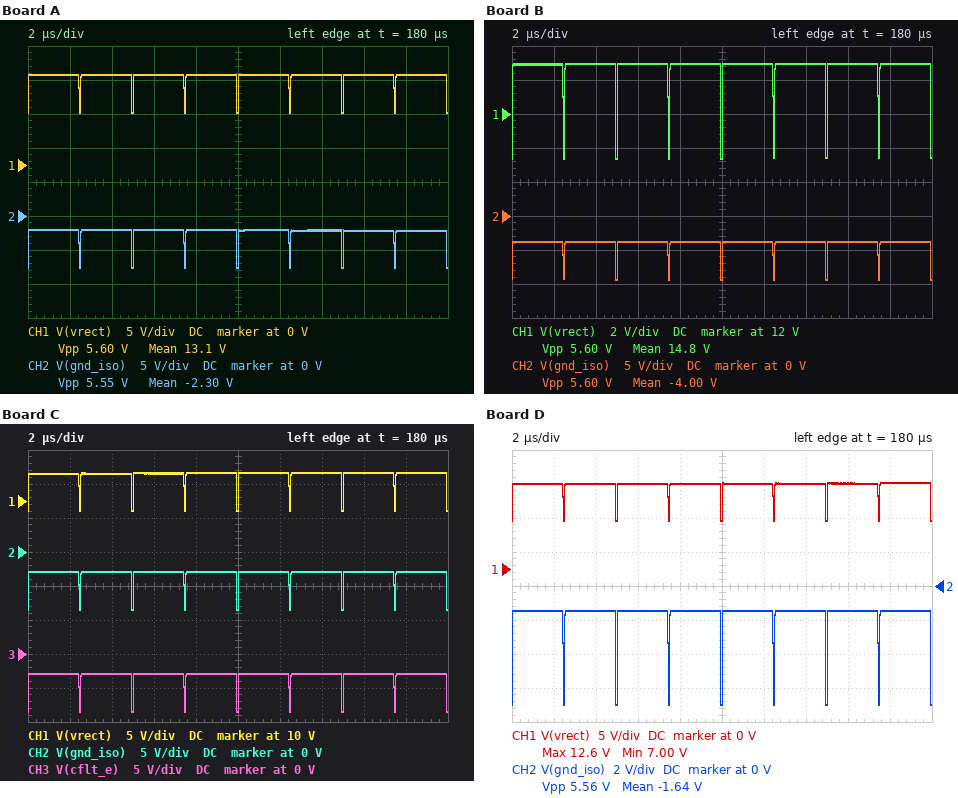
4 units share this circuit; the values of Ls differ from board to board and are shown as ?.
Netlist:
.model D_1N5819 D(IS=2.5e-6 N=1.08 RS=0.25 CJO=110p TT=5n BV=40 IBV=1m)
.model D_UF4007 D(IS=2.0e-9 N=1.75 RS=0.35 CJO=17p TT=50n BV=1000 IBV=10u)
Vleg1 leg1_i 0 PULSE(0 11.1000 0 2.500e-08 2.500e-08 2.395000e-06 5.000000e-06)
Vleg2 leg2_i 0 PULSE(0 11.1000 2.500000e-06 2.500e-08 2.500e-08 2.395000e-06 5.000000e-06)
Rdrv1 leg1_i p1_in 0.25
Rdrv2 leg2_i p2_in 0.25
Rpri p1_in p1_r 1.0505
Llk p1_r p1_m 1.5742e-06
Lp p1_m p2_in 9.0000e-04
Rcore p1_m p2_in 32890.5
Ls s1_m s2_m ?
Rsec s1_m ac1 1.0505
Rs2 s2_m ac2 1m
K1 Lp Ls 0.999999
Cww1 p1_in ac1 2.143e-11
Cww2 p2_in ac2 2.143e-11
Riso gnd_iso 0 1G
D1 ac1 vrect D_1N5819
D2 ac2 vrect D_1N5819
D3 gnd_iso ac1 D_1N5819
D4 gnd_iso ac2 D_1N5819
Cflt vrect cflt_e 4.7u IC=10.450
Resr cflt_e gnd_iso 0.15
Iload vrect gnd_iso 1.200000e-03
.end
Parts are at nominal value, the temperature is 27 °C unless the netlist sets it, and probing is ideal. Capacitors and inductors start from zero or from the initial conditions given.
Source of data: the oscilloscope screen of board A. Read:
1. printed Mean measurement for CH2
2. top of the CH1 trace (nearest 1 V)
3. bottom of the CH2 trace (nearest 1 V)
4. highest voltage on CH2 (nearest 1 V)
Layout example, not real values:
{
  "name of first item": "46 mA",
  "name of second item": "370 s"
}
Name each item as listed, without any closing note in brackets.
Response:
{
  "printed Mean measurement for CH2": "-2.30 V",
  "top of the CH1 trace": "13 V",
  "bottom of the CH2 trace": "-8 V",
  "highest voltage on CH2": "-2 V"
}
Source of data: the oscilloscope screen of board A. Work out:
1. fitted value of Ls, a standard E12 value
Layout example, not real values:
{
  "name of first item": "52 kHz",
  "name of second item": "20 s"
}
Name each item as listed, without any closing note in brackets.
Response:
{
  "fitted value of Ls, a standard E12 value": "1.8 mH"
}
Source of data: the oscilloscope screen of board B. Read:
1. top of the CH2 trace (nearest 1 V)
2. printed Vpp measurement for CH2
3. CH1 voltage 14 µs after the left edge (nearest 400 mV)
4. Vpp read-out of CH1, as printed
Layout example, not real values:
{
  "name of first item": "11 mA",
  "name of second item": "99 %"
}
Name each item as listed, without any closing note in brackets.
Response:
{
  "top of the CH2 trace": "-4 V",
  "printed Vpp measurement for CH2": "5.60 V",
  "CH1 voltage 14 µs after the left edge": "14.8 V",
  "Vpp read-out of CH1, as printed": "5.60 V"
}
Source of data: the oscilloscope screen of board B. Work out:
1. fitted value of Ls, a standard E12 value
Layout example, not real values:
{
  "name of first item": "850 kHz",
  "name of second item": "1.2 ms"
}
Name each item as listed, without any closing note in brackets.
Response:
{
  "fitted value of Ls, a standard E12 value": "2.7 mH"
}
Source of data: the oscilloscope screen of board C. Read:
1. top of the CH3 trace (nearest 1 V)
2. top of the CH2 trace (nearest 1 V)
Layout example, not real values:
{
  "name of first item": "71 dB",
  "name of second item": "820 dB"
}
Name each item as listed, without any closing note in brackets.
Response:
{
  "top of the CH3 trace": "-3 V",
  "top of the CH2 trace": "-3 V"
}
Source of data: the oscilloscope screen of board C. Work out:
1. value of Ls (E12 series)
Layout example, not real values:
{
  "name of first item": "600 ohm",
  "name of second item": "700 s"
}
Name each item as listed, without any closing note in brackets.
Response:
{
  "value of Ls": "2.2 mH"
}
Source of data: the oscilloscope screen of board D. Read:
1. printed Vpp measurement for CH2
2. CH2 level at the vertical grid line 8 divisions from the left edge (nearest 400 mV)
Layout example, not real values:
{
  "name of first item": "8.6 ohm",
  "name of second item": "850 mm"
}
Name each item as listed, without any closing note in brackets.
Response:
{
  "printed Vpp measurement for CH2": "5.56 V",
  "CH2 level at the vertical grid line 8 divisions from the left edge": "-1.6 V"
}
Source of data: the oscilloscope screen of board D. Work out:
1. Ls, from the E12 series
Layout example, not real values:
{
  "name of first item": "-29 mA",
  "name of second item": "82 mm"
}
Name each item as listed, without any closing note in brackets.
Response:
{
  "Ls, from the E12 series": "1.5 mH"
}
